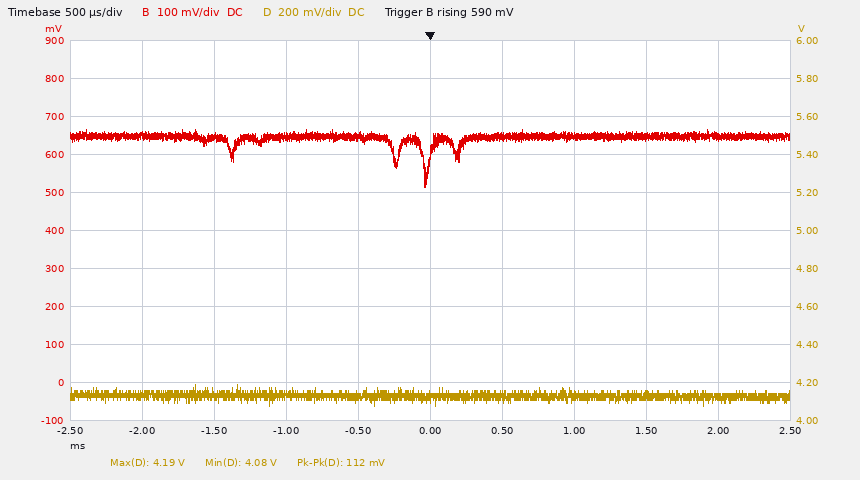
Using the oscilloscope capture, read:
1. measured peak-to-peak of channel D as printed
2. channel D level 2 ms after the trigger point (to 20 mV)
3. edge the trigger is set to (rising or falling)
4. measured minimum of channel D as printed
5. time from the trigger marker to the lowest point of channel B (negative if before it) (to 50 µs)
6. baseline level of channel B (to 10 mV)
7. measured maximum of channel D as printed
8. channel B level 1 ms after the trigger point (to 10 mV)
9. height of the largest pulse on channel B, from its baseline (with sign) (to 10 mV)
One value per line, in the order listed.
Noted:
112 mV
4.12 V
rising
4.08 V
-50 µs
650 mV
4.19 V
650 mV
-130 mV
